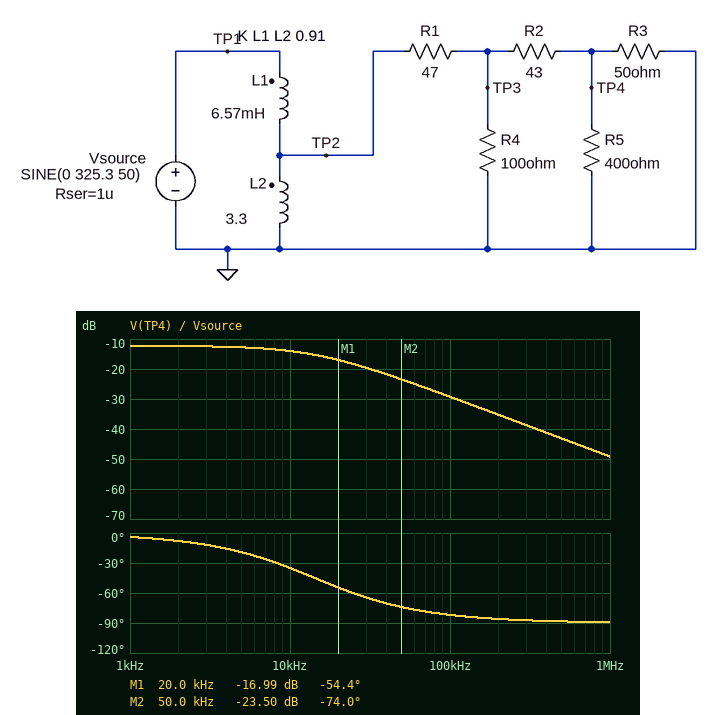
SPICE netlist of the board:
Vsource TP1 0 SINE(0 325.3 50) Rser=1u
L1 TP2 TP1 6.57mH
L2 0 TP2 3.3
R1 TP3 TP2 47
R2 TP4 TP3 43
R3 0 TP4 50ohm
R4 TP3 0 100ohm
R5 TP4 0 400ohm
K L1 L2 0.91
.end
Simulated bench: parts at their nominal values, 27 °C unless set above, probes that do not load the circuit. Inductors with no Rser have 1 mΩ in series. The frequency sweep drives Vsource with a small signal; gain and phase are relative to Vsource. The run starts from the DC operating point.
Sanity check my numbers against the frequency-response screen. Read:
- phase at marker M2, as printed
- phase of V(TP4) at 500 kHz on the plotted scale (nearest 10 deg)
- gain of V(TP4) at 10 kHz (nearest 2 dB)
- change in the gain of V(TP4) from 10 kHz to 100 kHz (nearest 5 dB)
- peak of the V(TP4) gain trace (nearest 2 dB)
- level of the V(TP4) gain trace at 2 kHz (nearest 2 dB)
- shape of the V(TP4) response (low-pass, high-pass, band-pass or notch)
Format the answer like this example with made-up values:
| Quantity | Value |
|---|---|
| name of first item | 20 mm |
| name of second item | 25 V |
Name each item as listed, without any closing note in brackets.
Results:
| Quantity | Value |
|---|---|
| phase at marker M2, as printed | -74.0 deg |
| phase of V(TP4) at 500 kHz on the plotted scale | -90 deg |
| gain of V(TP4) at 10 kHz | -14 dB |
| change in the gain of V(TP4) from 10 kHz to 100 kHz | -15 dB |
| peak of the V(TP4) gain trace | -12 dB |
| level of the V(TP4) gain trace at 2 kHz | -12 dB |
| shape of the V(TP4) response | low-pass |
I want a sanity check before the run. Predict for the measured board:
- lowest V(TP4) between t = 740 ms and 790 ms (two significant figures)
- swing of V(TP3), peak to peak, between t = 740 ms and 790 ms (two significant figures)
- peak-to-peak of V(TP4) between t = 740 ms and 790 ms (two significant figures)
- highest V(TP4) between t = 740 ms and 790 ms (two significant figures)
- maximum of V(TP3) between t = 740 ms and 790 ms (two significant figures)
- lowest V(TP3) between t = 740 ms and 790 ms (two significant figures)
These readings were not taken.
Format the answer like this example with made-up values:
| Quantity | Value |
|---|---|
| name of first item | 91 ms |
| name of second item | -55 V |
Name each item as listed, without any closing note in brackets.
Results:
| Quantity | Value |
|---|---|
| lowest V(TP4) between t = 740 ms and 790 ms | -79 V |
| swing of V(TP3), peak to peak, between t = 740 ms and 790 ms | 310 V |
| peak-to-peak of V(TP4) between t = 740 ms and 790 ms | 160 V |
| highest V(TP4) between t = 740 ms and 790 ms | 79 V |
| maximum of V(TP3) between t = 740 ms and 790 ms | 160 V |
| lowest V(TP3) between t = 740 ms and 790 ms | -160 V |
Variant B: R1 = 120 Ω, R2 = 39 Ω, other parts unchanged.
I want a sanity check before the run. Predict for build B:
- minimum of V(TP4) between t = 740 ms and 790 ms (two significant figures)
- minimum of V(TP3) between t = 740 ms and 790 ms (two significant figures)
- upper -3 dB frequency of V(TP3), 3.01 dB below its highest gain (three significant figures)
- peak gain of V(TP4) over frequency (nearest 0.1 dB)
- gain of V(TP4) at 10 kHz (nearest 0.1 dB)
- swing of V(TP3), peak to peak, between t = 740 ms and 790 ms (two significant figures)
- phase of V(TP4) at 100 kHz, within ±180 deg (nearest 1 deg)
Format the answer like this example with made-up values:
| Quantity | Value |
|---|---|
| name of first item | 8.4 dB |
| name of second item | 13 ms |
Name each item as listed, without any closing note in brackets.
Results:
| Quantity | Value |
|---|---|
| minimum of V(TP4) between t = 740 ms and 790 ms | -46 V |
| minimum of V(TP3) between t = 740 ms and 790 ms | -86 V |
| upper -3 dB frequency of V(TP3), 3.01 dB below its highest gain | 25.3 kHz |
| peak gain of V(TP4) over frequency | -17.0 dB |
| gain of V(TP4) at 10 kHz | -17.7 dB |
| swing of V(TP3), peak to peak, between t = 740 ms and 790 ms | 170 V |
| phase of V(TP4) at 100 kHz, within ±180 deg | -76 deg |
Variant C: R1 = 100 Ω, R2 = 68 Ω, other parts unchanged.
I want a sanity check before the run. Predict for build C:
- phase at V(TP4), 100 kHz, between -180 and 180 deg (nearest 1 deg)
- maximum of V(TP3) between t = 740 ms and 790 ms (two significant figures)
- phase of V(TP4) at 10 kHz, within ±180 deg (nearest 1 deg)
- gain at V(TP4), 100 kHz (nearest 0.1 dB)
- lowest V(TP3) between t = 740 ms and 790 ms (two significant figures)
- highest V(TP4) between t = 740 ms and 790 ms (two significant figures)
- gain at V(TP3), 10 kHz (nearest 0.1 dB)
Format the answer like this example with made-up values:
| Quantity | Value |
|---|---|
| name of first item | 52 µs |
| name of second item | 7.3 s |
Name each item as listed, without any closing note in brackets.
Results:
| Quantity | Value |
|---|---|
| phase at V(TP4), 100 kHz, between -180 and 180 deg | -77 deg |
| maximum of V(TP3) between t = 740 ms and 790 ms | 110 V |
| phase of V(TP4) at 10 kHz, within ±180 deg | -23 deg |
| gain at V(TP4), 100 kHz | -30.5 dB |
| lowest V(TP3) between t = 740 ms and 790 ms | -110 V |
| highest V(TP4) between t = 740 ms and 790 ms | 43 V |
| gain at V(TP3), 10 kHz | -10.3 dB |
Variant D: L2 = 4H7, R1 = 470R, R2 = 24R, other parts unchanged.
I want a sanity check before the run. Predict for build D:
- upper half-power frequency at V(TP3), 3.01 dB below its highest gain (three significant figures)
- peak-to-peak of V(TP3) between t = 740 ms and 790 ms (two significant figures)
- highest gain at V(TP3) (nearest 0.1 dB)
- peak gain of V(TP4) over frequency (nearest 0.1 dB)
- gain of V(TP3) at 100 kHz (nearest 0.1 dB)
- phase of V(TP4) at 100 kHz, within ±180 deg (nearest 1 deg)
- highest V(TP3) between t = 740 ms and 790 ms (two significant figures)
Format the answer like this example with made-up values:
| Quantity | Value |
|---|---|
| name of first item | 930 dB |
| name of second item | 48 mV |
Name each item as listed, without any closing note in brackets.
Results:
| Quantity | Value |
|---|---|
| upper half-power frequency at V(TP3), 3.01 dB below its highest gain | 77.0 kHz |
| peak-to-peak of V(TP3) between t = 740 ms and 790 ms | 50 V |
| highest gain at V(TP3) | -22.3 dB |
| peak gain of V(TP4) over frequency | -26.0 dB |
| gain of V(TP3) at 100 kHz | -26.6 dB |
| phase of V(TP4) at 100 kHz, within ±180 deg | -52 deg |
| highest V(TP3) between t = 740 ms and 790 ms | 25 V |
